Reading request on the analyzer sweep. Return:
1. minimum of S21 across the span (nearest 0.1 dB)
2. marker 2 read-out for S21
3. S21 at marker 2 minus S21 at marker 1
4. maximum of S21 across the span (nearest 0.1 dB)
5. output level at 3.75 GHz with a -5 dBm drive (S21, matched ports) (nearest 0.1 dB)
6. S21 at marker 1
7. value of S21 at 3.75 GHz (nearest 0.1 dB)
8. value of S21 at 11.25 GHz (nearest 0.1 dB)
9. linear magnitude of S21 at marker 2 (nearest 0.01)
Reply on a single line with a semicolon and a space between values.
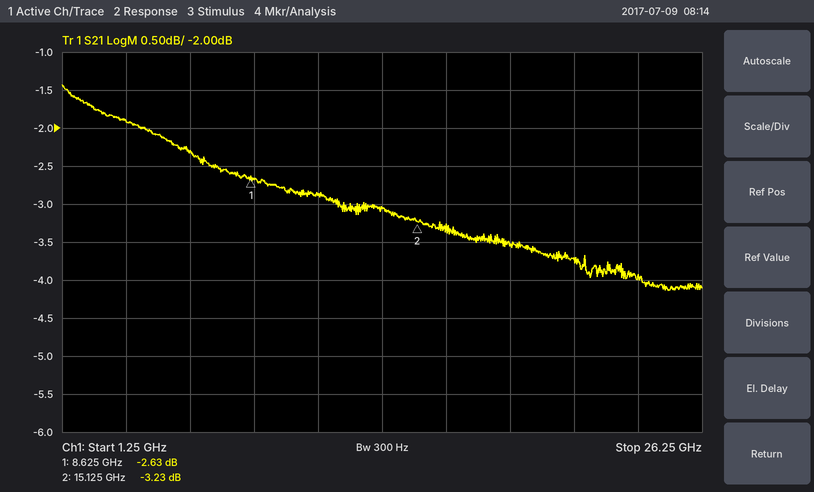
-4.1 dB; -3.23 dB; -0.60 dB; -1.4 dB; -6.9 dBm; -2.63 dB; -1.9 dB; -2.9 dB; 0.69
